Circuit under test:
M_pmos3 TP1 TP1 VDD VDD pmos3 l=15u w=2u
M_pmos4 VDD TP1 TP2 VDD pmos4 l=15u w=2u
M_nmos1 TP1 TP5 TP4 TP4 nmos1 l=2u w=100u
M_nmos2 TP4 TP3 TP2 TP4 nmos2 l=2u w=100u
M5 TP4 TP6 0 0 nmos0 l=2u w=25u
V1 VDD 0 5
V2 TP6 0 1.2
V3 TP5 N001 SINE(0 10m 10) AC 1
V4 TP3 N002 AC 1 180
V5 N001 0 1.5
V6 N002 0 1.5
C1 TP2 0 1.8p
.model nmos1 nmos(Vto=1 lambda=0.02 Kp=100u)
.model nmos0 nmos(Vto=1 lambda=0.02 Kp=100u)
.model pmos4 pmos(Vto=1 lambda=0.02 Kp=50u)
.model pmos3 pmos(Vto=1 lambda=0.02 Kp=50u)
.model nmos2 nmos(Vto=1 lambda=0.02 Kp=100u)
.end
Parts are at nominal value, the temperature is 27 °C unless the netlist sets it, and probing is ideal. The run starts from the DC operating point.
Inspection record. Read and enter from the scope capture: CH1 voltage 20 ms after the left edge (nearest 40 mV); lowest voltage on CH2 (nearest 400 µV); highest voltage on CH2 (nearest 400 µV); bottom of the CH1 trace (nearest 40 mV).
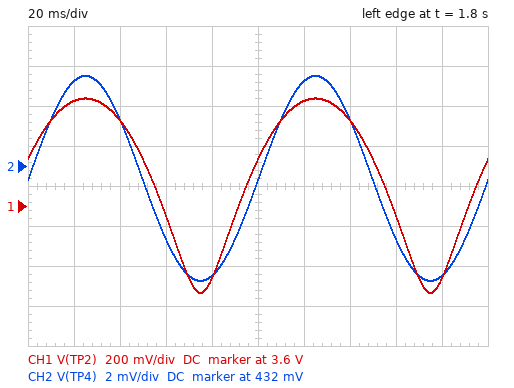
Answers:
4.12 V
426.4 mV
436.4 mV
3.16 V
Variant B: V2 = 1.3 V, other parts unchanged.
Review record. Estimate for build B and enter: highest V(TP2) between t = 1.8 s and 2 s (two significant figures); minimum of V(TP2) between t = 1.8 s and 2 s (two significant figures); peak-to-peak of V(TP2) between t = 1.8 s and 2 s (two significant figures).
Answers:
3.4 V
1.3 V
2.1 V
